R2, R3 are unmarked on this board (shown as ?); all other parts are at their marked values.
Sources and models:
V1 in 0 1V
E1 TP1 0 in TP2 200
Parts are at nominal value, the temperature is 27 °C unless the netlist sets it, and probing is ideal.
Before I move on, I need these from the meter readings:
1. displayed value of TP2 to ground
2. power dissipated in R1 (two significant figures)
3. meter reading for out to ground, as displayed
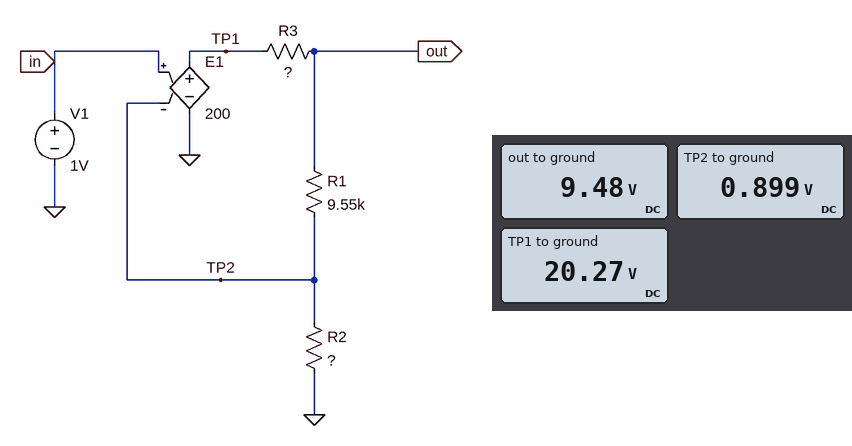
0.899 V
7.7 mW
9.48 V
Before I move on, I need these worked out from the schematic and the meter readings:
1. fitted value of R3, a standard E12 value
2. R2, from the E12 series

12 kΩ
1 kΩ
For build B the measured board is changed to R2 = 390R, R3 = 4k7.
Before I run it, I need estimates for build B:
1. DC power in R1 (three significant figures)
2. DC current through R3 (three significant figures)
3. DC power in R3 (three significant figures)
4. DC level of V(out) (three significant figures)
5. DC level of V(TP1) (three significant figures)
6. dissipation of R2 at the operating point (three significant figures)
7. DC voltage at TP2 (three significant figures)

44.5 mW
2.16 mA
21.9 mW
21.5 V
31.6 V
1.82 mW
842 mV
